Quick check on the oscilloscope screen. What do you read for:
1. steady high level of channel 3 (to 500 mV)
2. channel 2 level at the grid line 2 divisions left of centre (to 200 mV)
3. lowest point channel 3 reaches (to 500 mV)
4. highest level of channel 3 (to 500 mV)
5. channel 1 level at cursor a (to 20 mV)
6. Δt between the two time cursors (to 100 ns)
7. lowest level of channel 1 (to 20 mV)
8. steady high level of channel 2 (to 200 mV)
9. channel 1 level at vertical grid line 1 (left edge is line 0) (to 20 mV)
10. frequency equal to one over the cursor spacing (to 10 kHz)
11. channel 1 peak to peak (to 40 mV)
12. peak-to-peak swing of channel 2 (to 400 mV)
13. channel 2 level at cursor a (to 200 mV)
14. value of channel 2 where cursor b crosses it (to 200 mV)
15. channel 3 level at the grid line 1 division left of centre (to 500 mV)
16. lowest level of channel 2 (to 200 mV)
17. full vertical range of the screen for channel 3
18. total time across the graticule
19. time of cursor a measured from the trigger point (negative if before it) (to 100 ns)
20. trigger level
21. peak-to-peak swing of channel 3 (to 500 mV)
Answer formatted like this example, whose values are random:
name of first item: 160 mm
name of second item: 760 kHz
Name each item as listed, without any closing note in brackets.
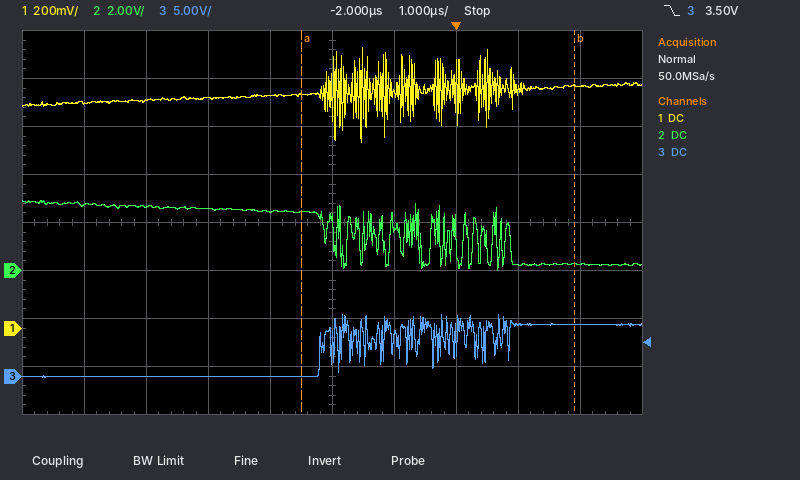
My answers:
steady high level of channel 3: 5.5 V
channel 2 level at the grid line 2 divisions left of centre: 2.6 V
lowest point channel 3 reaches: 0.0 V
highest level of channel 3: 6.5 V
channel 1 level at cursor a: 980 mV
Δt between the two time cursors: 4.4 µs
lowest level of channel 1: 780 mV
steady high level of channel 2: 2.6 V
channel 1 level at vertical grid line 1 (left edge is line 0): 940 mV
frequency equal to one over the cursor spacing: 230 kHz
channel 1 peak to peak: 400 mV
peak-to-peak swing of channel 2: 2.8 V
channel 2 level at cursor a: 2.4 V
value of channel 2 where cursor b crosses it: 200 mV
channel 3 level at the grid line 1 division left of centre: 0.0 V
lowest level of channel 2: 0.0 V
full vertical range of the screen for channel 3: 40 V
total time across the graticule: 10 µs
time of cursor a measured from the trigger point (negative if before it): -2.5 µs
trigger level: 3.50 V
peak-to-peak swing of channel 3: 6.5 V
